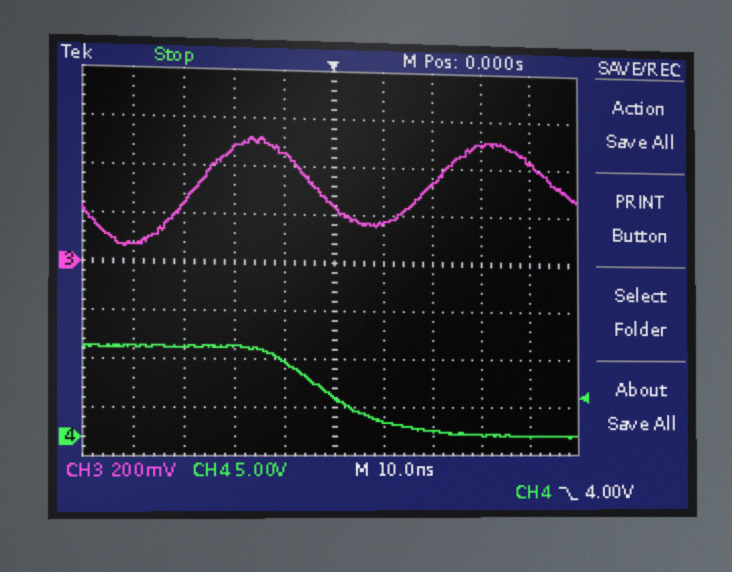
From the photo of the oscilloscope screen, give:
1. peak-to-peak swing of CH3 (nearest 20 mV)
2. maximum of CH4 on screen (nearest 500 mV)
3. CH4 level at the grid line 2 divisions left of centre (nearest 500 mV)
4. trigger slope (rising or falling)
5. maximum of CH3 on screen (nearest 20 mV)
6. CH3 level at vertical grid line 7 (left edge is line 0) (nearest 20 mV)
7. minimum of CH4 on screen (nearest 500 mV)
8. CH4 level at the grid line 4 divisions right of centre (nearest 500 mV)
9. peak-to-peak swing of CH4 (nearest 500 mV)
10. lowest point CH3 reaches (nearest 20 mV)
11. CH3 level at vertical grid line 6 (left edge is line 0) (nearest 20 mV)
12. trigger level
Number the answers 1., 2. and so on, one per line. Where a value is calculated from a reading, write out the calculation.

1. 520 mV − (60 mV) = 460 mV
2. 9.5 V
3. 9.5 V
4. falling
5. 520 mV
6. 340 mV
7. 0.0 V
8. 0.0 V
9. 9.5 V − (0.0 V) = 9.5 V
10. 60 mV
11. 160 mV
12. 4.00 V
